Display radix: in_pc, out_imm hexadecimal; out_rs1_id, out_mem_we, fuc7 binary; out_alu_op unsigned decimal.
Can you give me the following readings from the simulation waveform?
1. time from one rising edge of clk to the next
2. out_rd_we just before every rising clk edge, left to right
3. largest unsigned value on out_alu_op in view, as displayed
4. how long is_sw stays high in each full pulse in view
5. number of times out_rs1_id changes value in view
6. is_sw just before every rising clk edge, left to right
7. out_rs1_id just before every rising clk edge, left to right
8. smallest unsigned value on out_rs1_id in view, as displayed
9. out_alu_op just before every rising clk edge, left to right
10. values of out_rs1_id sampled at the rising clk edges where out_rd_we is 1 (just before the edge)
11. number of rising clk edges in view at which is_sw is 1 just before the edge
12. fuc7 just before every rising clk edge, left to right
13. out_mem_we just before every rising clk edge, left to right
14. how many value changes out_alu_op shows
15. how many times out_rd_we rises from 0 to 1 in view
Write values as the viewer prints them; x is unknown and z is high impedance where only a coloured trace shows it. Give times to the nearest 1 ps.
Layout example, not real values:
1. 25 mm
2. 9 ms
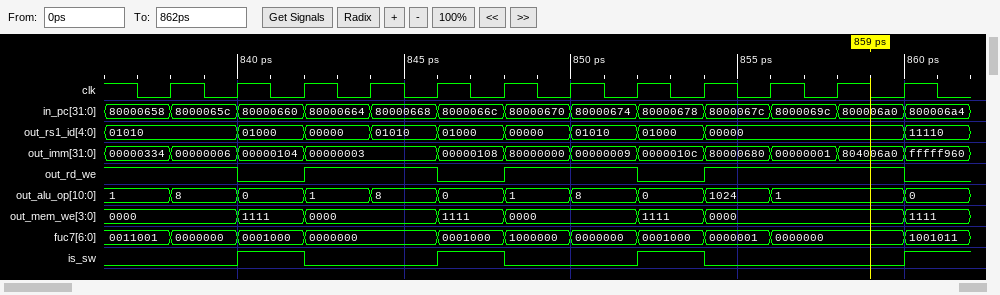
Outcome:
1. 2 ps
2. 1 1 0 1 1 0 1 1 0 1 1 1
3. 1024
4. 2 ps, 2 ps, 2 ps
5. 9
6. 0 0 1 0 0 1 0 0 1 0 0 0
7. 01010, 01010, 01000, 00000, 01010, 01000, 00000, 01010, 01000, 00000, 00000, 00000
8. 00000
9. 1, 8, 0, 1, 8, 0, 1, 8, 0, 1024, 1, 1
10. 01010, 01010, 00000, 01010, 00000, 01010, 00000, 00000, 00000
11. 3
12. 0011001, 0000000, 0001000, 0000000, 0000000, 0001000, 1000000, 0000000, 0001000, 0000001, 0000000, 0000000
13. 0000, 0000, 1111, 0000, 0000, 1111, 0000, 0000, 1111, 0000, 0000, 0000
14. 11
15. 3
